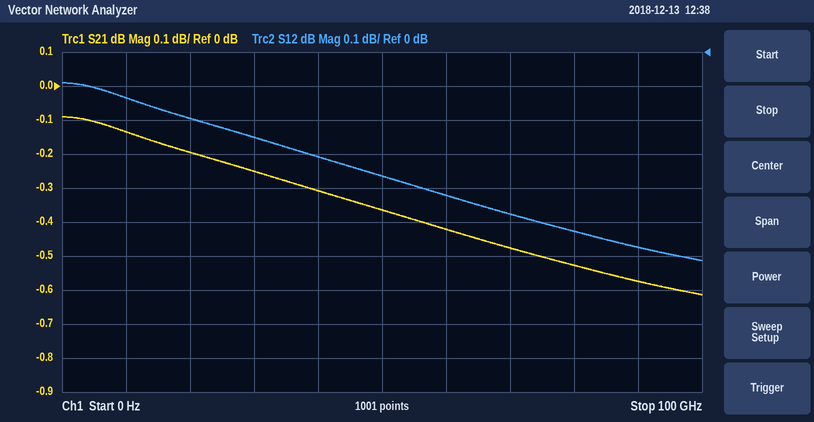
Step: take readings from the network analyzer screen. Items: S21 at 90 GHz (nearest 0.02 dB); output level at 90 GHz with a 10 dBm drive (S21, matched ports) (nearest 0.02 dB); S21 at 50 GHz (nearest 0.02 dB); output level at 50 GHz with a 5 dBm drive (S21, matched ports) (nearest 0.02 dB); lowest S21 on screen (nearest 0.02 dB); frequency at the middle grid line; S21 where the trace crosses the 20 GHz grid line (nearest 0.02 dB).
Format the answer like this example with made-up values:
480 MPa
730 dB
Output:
-0.58 dB
9.42 dBm
-0.36 dB
4.64 dBm
-0.62 dB
50 GHz
-0.20 dB
